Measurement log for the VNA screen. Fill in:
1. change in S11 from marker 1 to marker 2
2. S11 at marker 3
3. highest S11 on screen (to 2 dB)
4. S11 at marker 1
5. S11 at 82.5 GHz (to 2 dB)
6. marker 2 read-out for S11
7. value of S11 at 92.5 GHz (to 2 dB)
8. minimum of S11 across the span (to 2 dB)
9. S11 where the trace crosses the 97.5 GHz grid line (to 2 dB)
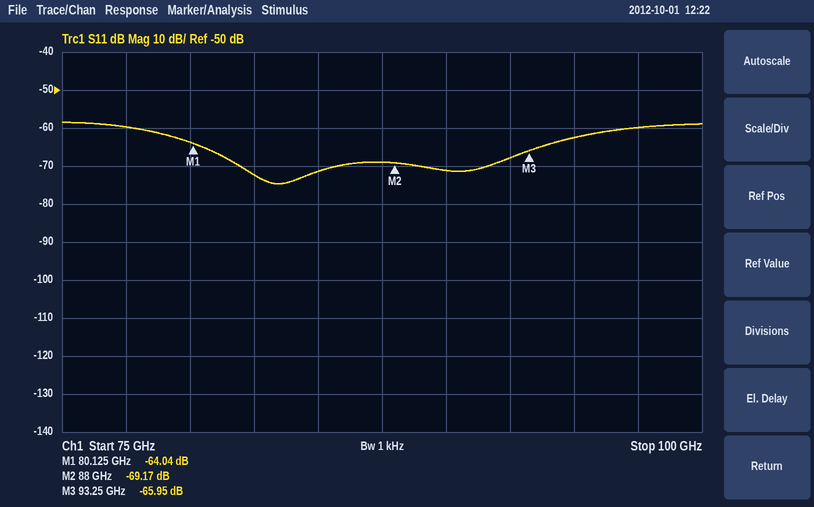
-5.13 dB
-65.95 dB
-58 dB
-64.04 dB
-72 dB
-69.17 dB
-68 dB
-74 dB
-60 dB
